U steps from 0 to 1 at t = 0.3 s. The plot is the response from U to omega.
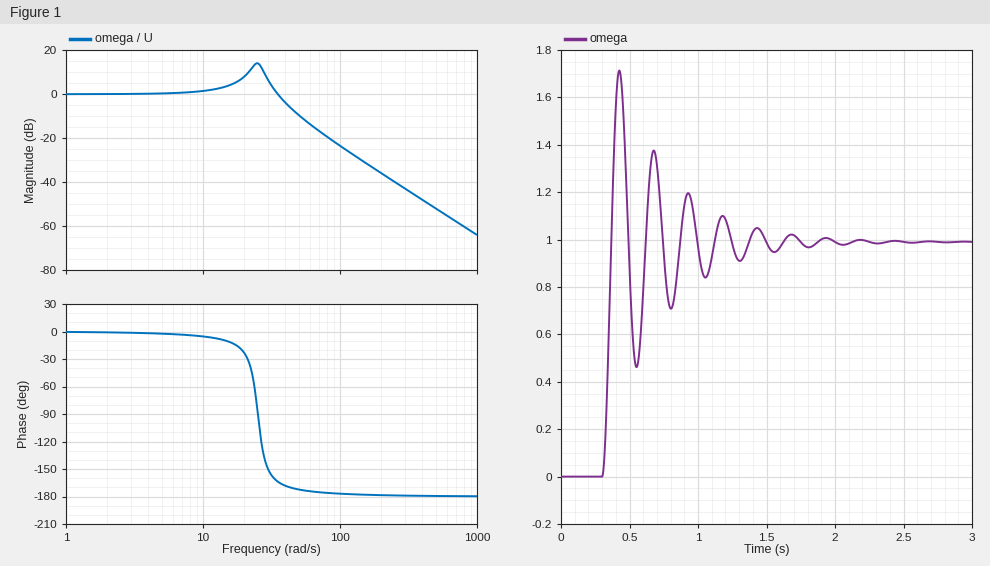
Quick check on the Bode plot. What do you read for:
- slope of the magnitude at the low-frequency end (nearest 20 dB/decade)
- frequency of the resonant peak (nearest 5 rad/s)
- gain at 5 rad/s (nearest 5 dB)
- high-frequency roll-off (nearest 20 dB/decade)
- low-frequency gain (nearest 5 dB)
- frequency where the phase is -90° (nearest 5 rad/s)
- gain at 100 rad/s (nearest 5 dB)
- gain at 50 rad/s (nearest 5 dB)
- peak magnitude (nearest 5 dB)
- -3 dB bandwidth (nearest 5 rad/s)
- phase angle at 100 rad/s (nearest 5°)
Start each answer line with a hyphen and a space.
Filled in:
- 0 dB/decade
- 25 rad/s
- 0 dB
- -40 dB/decade
- 0 dB
- 25 rad/s
- -25 dB
- -10 dB
- 15 dB
- 40 rad/s
- -175°
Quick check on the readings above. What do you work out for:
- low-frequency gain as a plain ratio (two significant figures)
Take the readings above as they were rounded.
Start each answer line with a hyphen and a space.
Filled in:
- 1.0
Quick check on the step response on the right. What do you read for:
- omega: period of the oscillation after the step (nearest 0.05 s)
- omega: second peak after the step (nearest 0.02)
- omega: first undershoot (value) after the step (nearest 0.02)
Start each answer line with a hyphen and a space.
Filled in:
- 0.25 s
- 1.38
- 0.46
